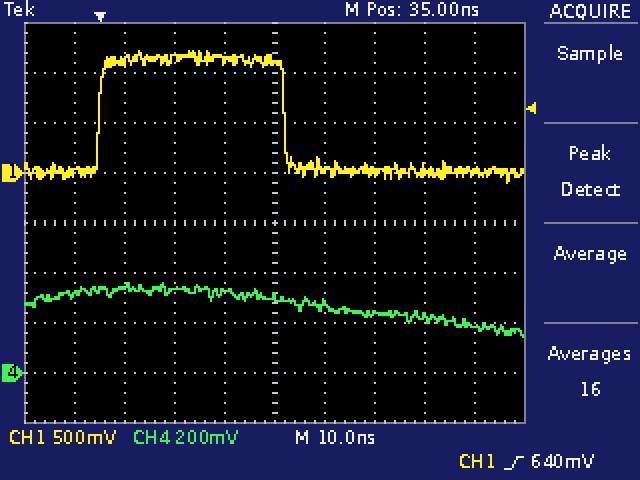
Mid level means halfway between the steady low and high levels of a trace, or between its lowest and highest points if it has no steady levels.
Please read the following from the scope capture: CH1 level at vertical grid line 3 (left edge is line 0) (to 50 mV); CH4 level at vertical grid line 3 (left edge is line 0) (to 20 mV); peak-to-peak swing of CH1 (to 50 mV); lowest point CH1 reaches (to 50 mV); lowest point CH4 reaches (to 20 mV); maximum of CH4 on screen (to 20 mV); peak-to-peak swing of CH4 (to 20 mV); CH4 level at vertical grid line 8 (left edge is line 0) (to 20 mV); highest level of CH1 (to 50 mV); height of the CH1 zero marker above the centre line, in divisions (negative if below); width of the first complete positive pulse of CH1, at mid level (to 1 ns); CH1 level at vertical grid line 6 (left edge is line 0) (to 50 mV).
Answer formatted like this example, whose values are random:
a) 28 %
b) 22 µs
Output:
a) 1.15 V
b) 340 mV
c) 1.30 V
d) -100 mV
e) 140 mV
f) 360 mV
g) 220 mV
h) 220 mV
i) 1.20 V
j) +1.0 div
k) 37 ns
l) 50 mV
